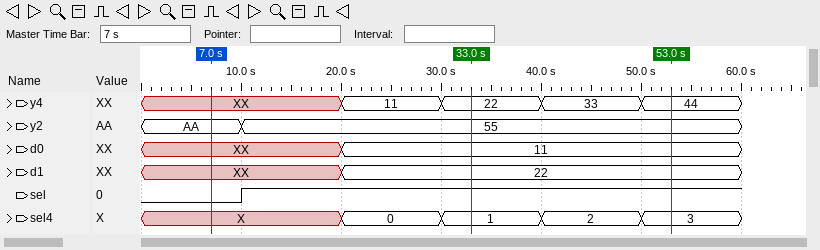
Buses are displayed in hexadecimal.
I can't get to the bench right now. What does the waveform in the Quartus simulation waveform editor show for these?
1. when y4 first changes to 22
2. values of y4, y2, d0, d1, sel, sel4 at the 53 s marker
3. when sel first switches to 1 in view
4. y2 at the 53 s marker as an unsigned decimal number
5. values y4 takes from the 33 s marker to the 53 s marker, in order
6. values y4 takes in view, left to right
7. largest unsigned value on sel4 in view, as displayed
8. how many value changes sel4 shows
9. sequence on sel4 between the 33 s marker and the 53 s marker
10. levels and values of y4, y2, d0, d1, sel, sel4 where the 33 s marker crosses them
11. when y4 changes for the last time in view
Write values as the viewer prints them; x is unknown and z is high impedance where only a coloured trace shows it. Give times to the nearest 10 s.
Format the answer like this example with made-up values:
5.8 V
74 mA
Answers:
30 s
y4=44, y2=55, d0=11, d1=22, sel=1, sel4=3
10 s
85
22, 33, 44
XX, 11, 22, 33, 44
3
4
1, 2, 3
y4=22, y2=55, d0=11, d1=22, sel=1, sel4=1
50 s
